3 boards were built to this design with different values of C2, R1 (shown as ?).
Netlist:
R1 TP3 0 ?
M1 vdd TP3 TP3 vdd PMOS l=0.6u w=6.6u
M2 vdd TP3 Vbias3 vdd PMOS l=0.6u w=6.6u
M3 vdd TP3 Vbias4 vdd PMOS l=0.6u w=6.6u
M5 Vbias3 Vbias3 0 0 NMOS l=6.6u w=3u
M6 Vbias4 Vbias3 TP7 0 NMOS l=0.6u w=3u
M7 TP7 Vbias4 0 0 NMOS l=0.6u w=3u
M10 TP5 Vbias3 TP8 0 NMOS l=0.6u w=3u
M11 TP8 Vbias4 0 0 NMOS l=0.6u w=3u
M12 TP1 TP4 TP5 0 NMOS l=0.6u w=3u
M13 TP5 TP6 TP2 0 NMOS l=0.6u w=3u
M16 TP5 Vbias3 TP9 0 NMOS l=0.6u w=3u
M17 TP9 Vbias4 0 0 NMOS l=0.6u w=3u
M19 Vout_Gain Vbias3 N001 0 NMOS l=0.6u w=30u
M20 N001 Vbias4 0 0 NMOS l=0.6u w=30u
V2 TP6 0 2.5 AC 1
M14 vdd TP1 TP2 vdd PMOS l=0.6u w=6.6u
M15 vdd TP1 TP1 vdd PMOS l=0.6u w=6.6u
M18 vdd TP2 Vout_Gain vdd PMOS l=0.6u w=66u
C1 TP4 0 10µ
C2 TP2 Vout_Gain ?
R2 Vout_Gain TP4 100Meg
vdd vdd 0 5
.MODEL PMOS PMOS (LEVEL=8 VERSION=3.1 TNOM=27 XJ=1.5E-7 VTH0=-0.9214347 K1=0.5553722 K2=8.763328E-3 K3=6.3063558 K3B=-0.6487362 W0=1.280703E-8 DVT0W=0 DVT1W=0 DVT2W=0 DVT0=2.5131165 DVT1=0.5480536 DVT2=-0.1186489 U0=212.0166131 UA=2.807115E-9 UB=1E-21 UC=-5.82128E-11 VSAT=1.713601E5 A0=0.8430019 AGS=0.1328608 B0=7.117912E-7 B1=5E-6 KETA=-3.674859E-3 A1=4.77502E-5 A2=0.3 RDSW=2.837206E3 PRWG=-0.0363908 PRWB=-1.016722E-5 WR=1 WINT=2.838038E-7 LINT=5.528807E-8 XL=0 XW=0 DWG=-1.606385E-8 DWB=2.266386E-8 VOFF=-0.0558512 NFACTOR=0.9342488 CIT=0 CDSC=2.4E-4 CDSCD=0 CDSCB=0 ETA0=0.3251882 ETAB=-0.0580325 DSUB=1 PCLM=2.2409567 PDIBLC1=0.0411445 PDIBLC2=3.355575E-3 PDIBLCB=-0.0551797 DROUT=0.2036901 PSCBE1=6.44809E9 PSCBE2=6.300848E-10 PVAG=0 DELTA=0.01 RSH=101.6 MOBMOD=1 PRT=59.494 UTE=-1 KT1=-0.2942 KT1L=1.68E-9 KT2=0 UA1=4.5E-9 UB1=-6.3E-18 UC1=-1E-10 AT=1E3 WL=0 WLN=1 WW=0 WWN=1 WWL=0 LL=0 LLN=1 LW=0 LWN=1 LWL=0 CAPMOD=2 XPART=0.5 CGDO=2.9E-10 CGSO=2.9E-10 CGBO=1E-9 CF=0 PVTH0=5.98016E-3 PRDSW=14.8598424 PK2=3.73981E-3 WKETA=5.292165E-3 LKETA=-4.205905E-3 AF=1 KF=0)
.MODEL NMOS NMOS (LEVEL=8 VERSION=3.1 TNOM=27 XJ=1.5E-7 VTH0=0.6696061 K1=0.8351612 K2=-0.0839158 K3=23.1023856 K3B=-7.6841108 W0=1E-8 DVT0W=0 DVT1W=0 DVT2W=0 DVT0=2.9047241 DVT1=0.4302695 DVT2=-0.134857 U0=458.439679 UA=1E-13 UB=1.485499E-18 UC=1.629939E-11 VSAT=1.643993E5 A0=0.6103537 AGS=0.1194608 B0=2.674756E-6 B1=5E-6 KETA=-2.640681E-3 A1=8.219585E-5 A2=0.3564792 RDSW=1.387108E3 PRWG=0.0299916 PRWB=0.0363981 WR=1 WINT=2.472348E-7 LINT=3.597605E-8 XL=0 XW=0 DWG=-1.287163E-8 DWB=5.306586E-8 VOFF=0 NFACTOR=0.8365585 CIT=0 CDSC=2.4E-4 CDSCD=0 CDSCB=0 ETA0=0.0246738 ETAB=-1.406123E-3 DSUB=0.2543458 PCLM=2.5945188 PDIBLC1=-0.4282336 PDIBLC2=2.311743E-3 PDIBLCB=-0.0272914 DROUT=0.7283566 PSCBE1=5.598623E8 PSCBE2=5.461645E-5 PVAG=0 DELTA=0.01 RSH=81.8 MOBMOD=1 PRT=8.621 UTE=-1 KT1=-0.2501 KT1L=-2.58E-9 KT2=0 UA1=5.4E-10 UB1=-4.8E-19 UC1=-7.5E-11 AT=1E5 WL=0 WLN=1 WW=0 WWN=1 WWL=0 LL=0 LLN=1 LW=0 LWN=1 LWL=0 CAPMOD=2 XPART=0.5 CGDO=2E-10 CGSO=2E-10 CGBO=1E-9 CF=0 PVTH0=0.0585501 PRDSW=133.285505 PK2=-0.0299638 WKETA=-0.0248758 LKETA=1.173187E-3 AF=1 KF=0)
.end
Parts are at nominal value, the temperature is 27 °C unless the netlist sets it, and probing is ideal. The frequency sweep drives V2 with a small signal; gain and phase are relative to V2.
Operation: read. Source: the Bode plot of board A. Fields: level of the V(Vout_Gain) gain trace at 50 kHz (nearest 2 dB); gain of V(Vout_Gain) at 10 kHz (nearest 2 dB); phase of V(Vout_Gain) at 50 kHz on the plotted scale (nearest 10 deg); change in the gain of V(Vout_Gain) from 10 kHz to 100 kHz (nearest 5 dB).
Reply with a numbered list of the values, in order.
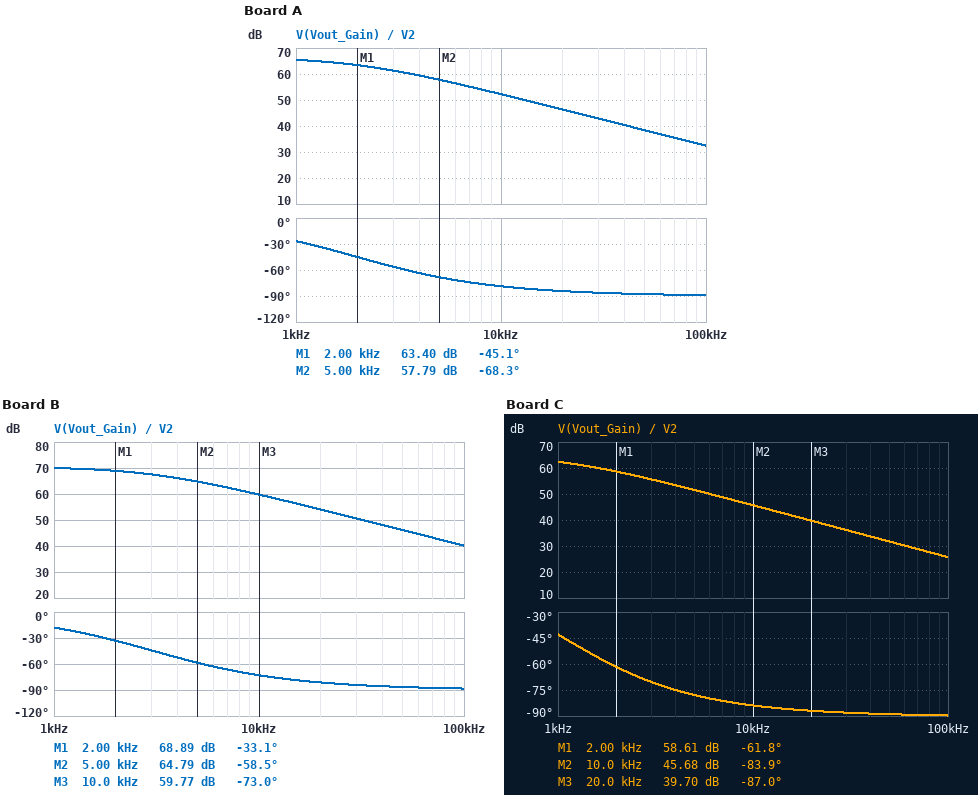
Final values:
1. 38 dB
2. 52 dB
3. -90 deg
4. -20 dB
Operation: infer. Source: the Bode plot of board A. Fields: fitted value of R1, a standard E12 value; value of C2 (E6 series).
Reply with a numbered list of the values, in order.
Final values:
1. 120 kΩ
2. 15 pF
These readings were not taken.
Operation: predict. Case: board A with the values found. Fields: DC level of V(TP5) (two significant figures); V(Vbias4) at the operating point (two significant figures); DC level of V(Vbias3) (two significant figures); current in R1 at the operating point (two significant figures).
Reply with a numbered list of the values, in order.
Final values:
1. 1.1 V
2. 1.1 V
3. 1.7 V
4. 31 µA
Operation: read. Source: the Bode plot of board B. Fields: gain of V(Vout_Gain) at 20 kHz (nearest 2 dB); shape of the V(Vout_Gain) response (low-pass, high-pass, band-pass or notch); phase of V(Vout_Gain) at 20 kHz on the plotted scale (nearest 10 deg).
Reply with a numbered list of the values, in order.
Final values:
1. 54 dB
2. low-pass
3. -80 deg
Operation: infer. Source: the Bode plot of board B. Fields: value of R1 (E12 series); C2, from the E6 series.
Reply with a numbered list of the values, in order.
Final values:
1. 270 kΩ
2. 4.7 pF
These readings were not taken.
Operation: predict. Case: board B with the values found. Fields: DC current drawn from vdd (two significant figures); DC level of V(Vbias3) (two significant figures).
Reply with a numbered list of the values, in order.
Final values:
1. 550 µA
2. 1.3 V
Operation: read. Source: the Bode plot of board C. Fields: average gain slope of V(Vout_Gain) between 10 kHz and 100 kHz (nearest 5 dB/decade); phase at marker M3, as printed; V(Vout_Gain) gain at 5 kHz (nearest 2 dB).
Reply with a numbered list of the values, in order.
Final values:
1. -20 dB/decade
2. -87.0 deg
3. 52 dB
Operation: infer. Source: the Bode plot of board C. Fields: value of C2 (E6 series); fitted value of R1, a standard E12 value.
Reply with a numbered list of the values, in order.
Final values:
1. 33 pF
2. 100 kΩ
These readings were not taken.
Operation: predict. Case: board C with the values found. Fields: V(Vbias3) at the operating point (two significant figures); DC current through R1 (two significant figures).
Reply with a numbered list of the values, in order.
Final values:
1. 1.8 V
2. 37 µA
